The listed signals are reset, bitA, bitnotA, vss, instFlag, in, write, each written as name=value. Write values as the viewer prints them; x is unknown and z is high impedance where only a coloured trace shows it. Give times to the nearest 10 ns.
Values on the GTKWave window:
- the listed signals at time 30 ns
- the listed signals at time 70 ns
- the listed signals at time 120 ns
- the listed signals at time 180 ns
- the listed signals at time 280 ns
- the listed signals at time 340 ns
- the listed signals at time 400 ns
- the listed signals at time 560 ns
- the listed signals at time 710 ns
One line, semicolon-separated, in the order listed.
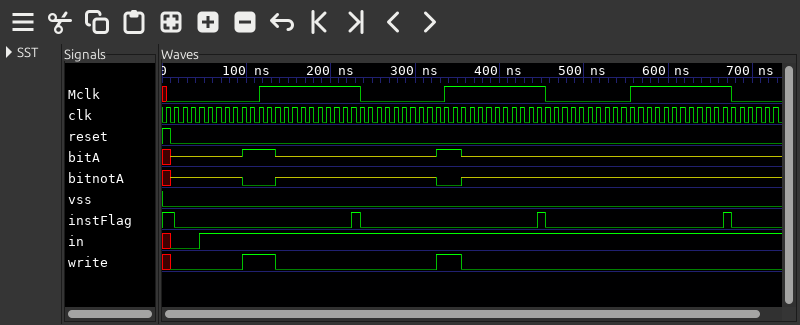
reset=0, bitA=z, bitnotA=z, vss=0, instFlag=0, in=0, write=0; reset=0, bitA=z, bitnotA=z, vss=0, instFlag=0, in=1, write=0; reset=0, bitA=1, bitnotA=0, vss=0, instFlag=0, in=1, write=1; reset=0, bitA=z, bitnotA=z, vss=0, instFlag=0, in=1, write=0; reset=0, bitA=z, bitnotA=z, vss=0, instFlag=0, in=1, write=0; reset=0, bitA=1, bitnotA=0, vss=0, instFlag=0, in=1, write=1; reset=0, bitA=z, bitnotA=z, vss=0, instFlag=0, in=1, write=0; reset=0, bitA=z, bitnotA=z, vss=0, instFlag=0, in=1, write=0; reset=0, bitA=z, bitnotA=z, vss=0, instFlag=0, in=1, write=0
